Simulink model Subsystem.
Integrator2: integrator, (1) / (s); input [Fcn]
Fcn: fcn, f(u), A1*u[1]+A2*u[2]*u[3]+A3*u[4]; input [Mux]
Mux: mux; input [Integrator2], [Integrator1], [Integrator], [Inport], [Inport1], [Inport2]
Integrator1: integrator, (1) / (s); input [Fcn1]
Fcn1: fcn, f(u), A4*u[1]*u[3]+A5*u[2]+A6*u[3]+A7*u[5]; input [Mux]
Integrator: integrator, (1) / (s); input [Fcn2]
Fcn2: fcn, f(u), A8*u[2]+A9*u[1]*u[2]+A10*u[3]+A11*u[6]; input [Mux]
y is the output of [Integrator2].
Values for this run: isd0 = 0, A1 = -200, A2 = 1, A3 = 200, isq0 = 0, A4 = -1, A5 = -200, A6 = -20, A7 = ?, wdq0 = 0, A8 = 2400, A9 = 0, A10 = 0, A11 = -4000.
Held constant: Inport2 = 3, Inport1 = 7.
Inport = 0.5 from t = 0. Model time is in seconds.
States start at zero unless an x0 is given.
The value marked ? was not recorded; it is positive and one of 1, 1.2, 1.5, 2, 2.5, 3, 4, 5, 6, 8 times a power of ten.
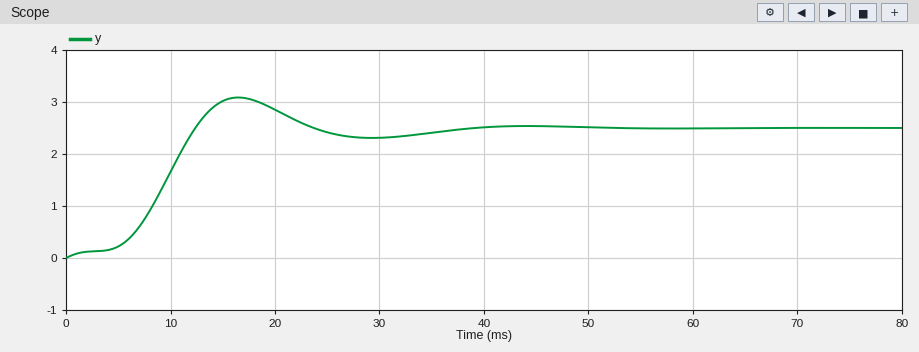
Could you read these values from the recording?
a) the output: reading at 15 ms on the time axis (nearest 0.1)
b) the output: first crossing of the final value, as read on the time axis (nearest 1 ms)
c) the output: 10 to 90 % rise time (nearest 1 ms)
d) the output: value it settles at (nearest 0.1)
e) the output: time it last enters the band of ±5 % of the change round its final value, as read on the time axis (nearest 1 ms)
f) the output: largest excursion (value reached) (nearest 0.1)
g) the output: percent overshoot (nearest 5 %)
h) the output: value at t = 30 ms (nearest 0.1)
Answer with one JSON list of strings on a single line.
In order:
["3.0", "12 ms", "6 ms", "2.5", "34 ms", "3.1", "25 %", "2.3"]
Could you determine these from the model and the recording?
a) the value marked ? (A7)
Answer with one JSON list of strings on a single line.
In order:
["400"]
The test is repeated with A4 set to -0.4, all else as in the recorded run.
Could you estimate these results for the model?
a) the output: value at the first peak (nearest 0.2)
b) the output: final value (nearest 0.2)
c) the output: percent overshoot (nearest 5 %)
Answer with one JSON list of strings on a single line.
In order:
["3.2", "2.6", "25 %"]
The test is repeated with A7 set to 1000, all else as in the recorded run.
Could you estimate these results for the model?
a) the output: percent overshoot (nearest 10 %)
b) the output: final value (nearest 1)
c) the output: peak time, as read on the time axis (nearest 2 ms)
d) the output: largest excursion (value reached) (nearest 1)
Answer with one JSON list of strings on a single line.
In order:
["90 %", "6", "12 ms", "12"]
